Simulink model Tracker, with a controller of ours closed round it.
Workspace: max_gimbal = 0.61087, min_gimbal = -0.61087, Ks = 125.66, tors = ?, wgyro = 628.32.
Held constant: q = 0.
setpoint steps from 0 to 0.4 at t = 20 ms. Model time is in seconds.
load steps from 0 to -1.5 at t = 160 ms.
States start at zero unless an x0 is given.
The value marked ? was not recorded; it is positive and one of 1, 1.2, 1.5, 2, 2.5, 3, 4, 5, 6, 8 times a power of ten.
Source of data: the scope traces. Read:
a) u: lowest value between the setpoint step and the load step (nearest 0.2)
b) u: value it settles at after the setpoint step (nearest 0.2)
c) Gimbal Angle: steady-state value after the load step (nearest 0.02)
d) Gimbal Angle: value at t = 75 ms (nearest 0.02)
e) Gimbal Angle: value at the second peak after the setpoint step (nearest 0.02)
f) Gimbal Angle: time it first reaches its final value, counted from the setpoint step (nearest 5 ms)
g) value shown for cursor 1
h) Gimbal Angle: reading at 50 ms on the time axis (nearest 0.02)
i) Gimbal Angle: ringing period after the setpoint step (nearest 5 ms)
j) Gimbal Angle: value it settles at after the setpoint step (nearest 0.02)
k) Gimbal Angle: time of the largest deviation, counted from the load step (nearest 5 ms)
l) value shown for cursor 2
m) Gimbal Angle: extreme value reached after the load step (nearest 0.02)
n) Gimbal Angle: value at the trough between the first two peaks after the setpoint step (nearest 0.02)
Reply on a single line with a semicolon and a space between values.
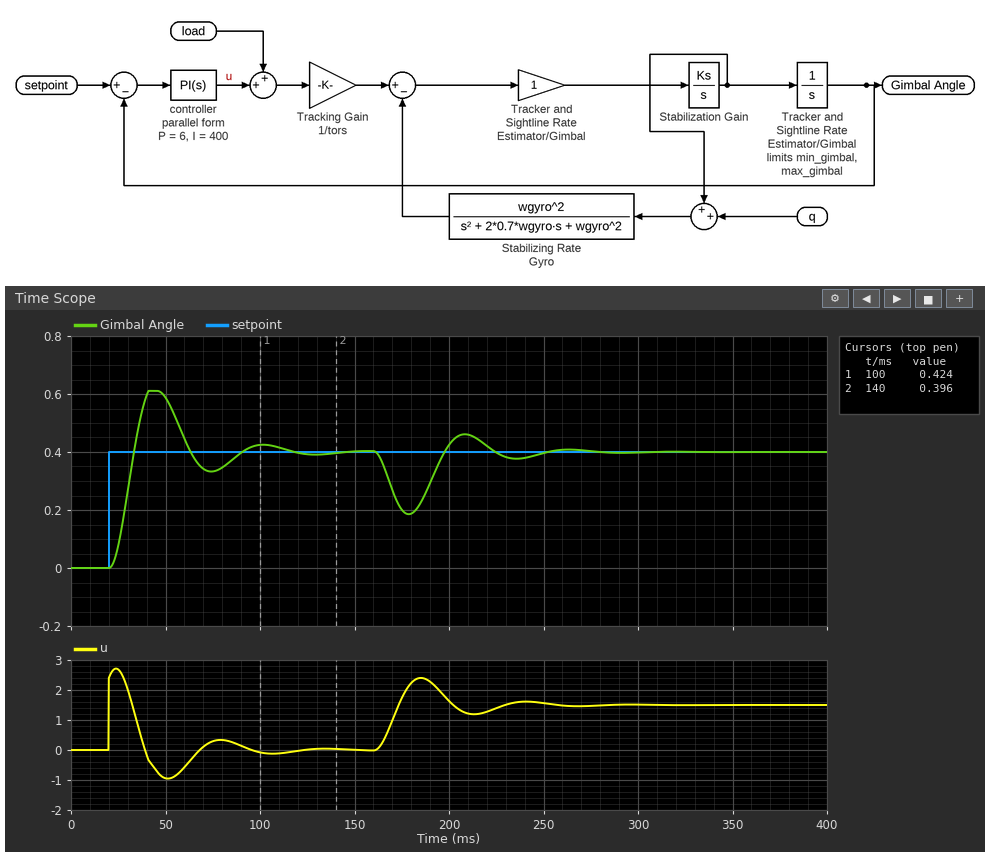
-1.0; 0.0; 0.40; 0.34; 0.42; 15 ms; 0.424; 0.58; 60 ms; 0.40; 20 ms; 0.396; 0.18; 0.34
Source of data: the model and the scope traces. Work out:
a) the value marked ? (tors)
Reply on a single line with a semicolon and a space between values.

0.05
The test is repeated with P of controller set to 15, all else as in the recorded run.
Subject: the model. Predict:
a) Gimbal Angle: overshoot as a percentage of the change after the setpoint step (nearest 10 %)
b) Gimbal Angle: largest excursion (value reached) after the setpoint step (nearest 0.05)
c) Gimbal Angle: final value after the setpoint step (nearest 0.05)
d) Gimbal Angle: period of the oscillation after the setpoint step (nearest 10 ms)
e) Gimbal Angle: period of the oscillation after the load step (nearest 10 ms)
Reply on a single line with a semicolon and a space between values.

50 %; 0.60; 0.40; 30 ms; 30 ms
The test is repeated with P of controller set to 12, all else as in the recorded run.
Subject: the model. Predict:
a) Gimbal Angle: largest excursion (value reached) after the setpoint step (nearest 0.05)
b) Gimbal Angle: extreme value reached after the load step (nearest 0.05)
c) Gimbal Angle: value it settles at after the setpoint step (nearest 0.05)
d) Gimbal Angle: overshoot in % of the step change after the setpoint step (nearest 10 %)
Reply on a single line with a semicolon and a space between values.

0.60; 0.25; 0.40; 50 %
